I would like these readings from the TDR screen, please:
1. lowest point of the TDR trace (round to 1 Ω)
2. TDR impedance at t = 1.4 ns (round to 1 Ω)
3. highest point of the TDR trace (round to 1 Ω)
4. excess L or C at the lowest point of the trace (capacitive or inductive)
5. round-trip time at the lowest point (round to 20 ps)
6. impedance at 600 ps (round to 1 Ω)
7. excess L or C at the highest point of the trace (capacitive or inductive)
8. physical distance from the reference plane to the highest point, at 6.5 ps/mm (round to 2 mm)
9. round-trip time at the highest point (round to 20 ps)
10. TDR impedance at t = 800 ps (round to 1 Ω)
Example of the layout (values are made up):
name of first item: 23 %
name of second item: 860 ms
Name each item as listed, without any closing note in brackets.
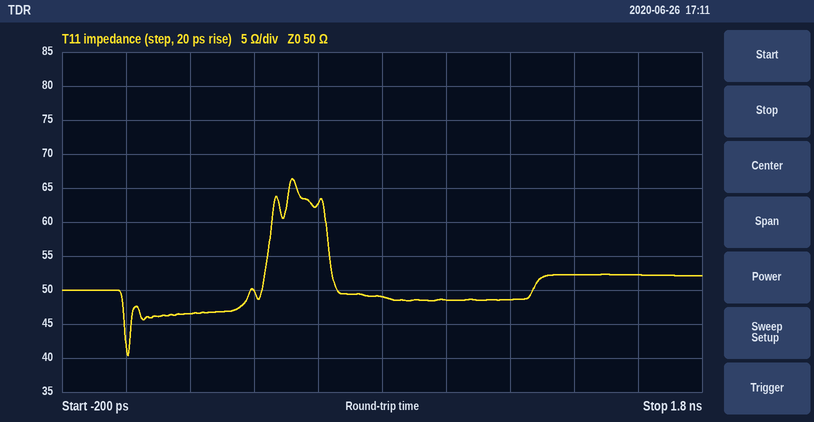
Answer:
lowest point of the TDR trace: 40 Ω
TDR impedance at t = 1.4 ns: 52 Ω
highest point of the TDR trace: 66 Ω
excess L or C at the lowest point of the trace: capacitive
round-trip time at the lowest point: 0 ps
impedance at 600 ps: 63 Ω
excess L or C at the highest point of the trace: inductive
physical distance from the reference plane to the highest point, at 6.5 ps/mm: 40 mm
round-trip time at the highest point: 520 ps
TDR impedance at t = 800 ps: 49 Ω
